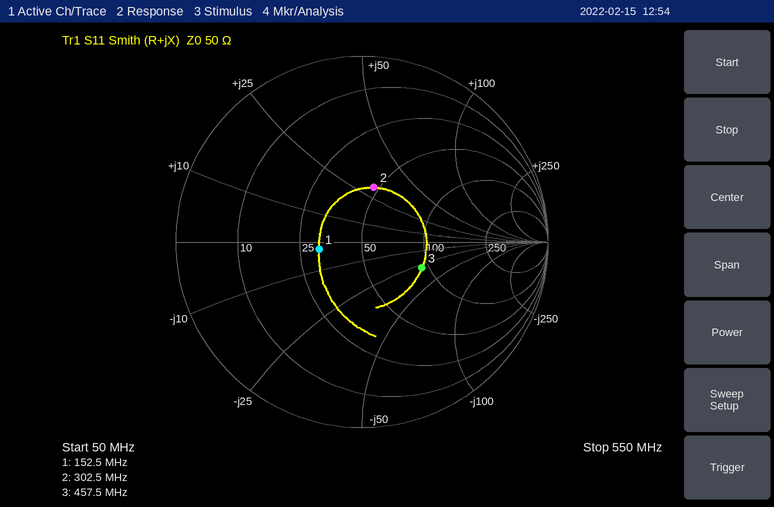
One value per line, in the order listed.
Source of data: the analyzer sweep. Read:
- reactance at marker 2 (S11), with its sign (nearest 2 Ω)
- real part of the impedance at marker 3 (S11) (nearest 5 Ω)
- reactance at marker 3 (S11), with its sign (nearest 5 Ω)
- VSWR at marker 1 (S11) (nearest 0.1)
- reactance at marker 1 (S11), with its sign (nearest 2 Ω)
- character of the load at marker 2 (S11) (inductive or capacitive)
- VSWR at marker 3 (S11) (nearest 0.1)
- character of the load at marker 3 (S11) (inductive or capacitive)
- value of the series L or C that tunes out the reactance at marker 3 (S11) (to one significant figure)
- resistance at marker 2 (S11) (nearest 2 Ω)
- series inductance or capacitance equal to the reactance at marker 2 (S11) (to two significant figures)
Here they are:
+30 Ω
90 Ω
-30 Ω
1.6
-2 Ω
inductive
2.1
capacitive
10 nH
48 Ω
16 nH
